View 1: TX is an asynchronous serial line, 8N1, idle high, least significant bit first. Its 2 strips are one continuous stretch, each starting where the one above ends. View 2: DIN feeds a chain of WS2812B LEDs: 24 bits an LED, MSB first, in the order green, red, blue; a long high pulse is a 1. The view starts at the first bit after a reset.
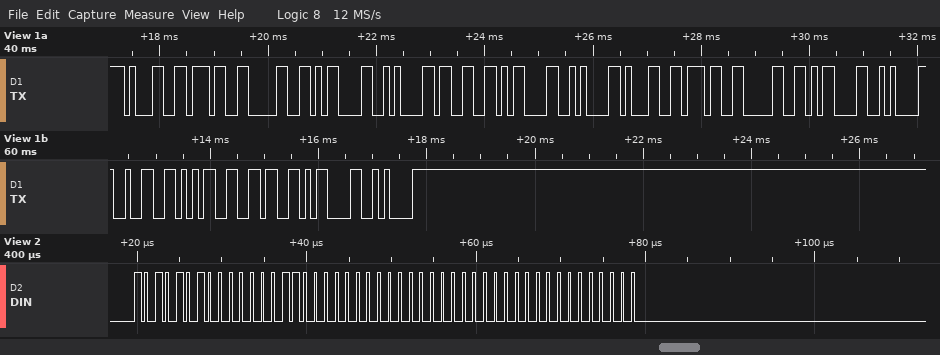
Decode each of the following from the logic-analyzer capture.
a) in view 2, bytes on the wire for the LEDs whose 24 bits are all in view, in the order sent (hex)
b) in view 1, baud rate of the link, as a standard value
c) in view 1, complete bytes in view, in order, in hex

AA 03 00 00 00 00
9600 baud
31 37 30 0D 0A 33 0D 0A 31 37 30 0D 0A 32 35 36 0D 0A
